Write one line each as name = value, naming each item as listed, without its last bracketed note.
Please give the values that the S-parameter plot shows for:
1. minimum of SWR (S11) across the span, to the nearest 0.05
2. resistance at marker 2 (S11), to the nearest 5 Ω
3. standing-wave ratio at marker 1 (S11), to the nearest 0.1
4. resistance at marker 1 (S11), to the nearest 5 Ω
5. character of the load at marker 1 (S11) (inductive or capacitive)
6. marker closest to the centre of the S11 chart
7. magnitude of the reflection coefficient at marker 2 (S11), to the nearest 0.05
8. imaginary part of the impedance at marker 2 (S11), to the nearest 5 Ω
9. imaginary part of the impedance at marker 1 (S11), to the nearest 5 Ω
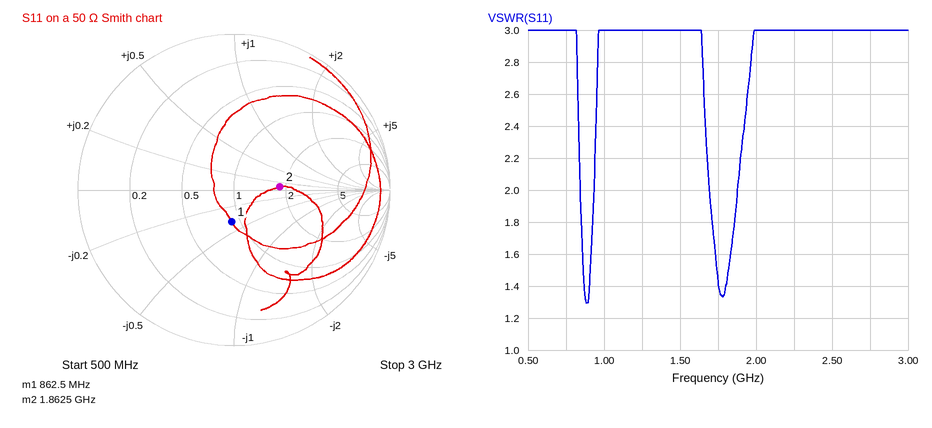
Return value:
minimum of SWR (S11) across the span, to the nearest 0.05 = 1.30
resistance at marker 2 (S11), to the nearest 5 Ω = 90 Ω
standing-wave ratio at marker 1 (S11), to the nearest 0.1 = 1.5
resistance at marker 1 (S11), to the nearest 5 Ω = 45 Ω
character of the load at marker 1 (S11) = capacitive
marker closest to the centre of the S11 chart = marker 1
magnitude of the reflection coefficient at marker 2 (S11), to the nearest 0.05 = 0.30
imaginary part of the impedance at marker 2 (S11), to the nearest 5 Ω = +5 Ω
imaginary part of the impedance at marker 1 (S11), to the nearest 5 Ω = -20 Ω
